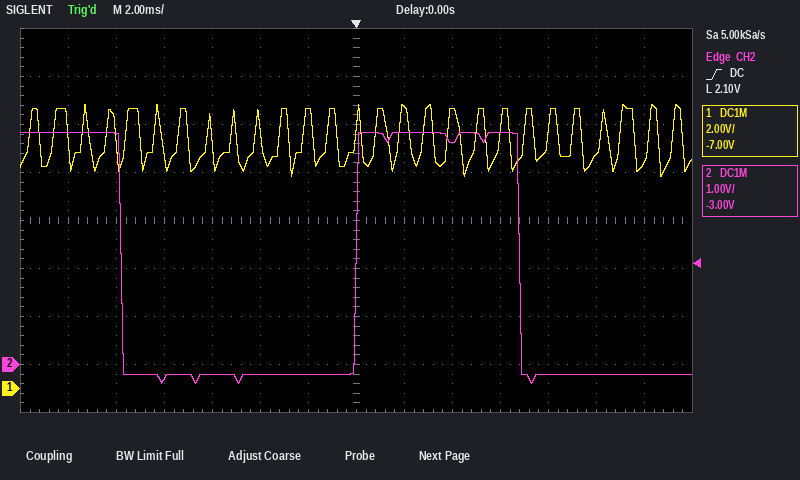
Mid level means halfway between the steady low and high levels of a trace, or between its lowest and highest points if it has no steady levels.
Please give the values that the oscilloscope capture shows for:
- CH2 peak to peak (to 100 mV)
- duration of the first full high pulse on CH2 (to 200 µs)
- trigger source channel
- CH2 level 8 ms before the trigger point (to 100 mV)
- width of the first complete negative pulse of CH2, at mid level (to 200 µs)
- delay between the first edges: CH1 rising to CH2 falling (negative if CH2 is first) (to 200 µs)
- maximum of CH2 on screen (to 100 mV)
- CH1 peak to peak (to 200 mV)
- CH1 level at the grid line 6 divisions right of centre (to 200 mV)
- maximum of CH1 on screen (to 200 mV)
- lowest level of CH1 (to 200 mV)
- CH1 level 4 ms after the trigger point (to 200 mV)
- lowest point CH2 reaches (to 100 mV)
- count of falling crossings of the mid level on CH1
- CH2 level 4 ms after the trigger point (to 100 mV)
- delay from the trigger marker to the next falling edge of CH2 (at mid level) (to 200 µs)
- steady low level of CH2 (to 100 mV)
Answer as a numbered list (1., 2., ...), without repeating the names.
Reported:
1. 5.2 V
2. 6.8 ms
3. CH2
4. -300 mV
5. 9.8 ms
6. +3.8 ms
7. 4.8 V
8. 3.0 V
9. 9.4 V
10. 11.8 V
11. 8.8 V
12. 11.6 V
13. -400 mV
14. 27
15. 4.6 V
16. 6.8 ms
17. -200 mV
